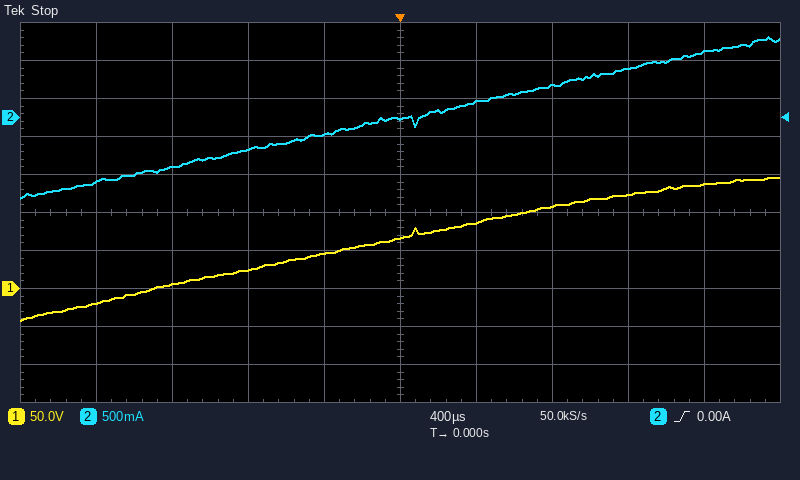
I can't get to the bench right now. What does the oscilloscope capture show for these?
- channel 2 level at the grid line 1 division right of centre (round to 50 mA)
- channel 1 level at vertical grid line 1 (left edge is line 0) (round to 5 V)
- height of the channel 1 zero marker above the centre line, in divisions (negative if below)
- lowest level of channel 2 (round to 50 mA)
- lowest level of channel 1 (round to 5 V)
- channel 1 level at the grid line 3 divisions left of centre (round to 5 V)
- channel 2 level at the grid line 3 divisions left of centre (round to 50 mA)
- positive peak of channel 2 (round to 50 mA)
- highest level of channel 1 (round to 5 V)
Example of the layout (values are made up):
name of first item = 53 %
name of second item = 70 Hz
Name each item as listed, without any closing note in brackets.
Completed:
channel 2 level at the grid line 1 division right of centre = 200 mA
channel 1 level at vertical grid line 1 (left edge is line 0) = -20 V
height of the channel 1 zero marker above the centre line, in divisions = -2.0 div
lowest level of channel 2 = -1.05 A
lowest level of channel 1 = -40 V
channel 1 level at the grid line 3 divisions left of centre = 5 V
channel 2 level at the grid line 3 divisions left of centre = -650 mA
positive peak of channel 2 = 1.05 A
highest level of channel 1 = 145 V
